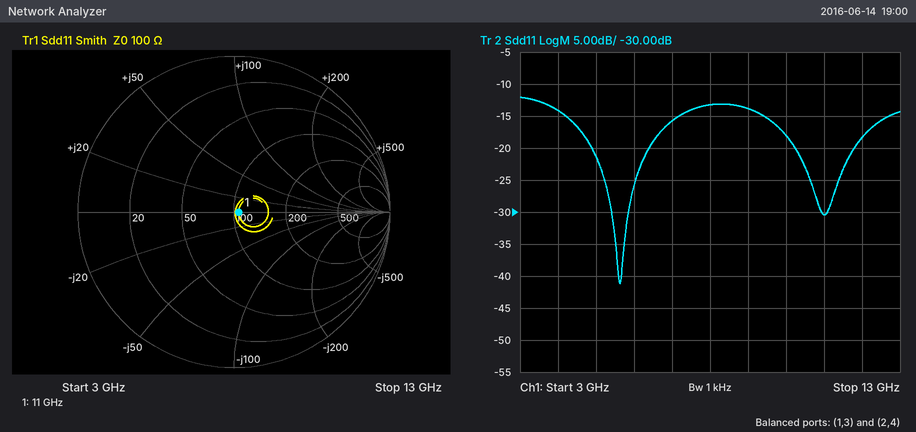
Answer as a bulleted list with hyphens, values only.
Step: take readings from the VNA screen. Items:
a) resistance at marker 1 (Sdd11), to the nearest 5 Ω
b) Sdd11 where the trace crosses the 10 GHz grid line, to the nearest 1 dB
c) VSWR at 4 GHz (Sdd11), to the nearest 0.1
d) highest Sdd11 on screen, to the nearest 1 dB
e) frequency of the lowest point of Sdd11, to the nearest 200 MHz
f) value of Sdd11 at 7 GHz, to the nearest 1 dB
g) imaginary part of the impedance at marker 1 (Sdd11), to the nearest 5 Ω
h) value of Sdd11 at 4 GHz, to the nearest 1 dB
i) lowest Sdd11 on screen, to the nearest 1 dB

- 105 Ω
- -18 dB
- 1.5
- -12 dB
- 5.6 GHz
- -16 dB
- 0 Ω
- -14 dB
- -41 dB
